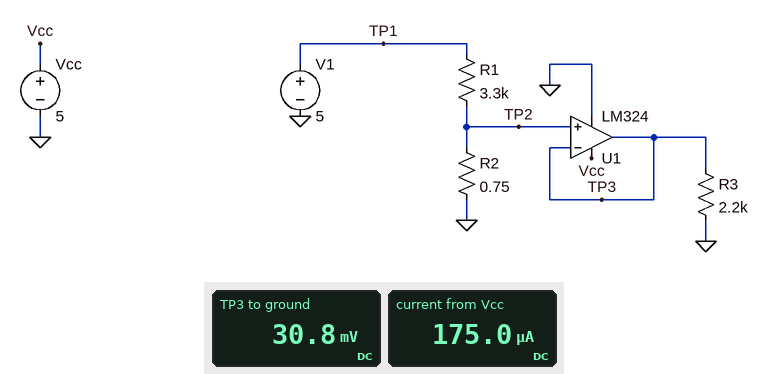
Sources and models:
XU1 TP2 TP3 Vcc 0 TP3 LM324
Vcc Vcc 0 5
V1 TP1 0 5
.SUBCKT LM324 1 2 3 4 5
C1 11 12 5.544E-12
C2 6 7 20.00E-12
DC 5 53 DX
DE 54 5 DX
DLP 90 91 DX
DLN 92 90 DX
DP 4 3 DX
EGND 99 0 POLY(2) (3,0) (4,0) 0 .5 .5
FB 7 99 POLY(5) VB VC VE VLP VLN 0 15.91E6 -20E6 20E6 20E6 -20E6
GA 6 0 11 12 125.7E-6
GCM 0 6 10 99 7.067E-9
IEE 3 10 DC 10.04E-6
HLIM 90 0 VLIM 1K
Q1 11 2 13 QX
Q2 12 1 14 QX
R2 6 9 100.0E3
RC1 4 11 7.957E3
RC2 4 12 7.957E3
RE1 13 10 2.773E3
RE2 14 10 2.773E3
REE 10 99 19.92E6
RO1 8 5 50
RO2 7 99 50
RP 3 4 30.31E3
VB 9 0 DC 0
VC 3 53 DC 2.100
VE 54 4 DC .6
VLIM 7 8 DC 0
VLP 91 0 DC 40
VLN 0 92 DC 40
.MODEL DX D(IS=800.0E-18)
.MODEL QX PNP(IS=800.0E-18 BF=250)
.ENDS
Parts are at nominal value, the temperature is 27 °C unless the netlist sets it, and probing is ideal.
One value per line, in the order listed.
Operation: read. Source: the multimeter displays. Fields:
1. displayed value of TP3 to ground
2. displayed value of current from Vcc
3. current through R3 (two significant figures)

30.8 mV
175.0 µA
14 µA
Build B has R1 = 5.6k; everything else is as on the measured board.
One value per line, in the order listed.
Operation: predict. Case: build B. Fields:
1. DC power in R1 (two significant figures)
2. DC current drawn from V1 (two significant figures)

4.5 mW
890 µA
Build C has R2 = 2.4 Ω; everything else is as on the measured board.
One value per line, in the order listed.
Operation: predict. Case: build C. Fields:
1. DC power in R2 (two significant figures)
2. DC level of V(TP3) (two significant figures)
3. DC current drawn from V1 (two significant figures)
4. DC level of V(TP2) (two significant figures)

5.5 µW
32 mV
1.5 mA
3.6 mV
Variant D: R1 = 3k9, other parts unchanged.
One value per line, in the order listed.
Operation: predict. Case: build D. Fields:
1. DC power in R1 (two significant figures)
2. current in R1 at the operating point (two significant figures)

6.4 mW
1.3 mA
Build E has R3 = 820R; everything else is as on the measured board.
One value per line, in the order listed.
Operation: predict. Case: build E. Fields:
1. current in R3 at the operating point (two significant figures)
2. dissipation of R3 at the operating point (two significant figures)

38 µA
1.2 µW
